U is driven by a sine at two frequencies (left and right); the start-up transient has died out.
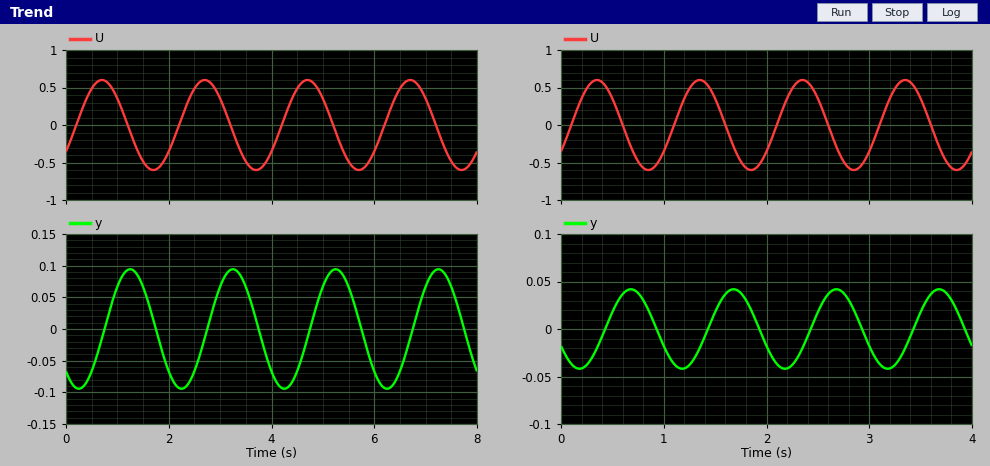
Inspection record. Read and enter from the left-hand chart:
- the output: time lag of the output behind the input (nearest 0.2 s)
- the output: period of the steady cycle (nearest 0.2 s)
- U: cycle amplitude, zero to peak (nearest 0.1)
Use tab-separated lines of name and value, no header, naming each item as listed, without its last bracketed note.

the output: time lag of the output behind the input	0.6 s
the output: period of the steady cycle	2.0 s
U: cycle amplitude, zero to peak	0.6
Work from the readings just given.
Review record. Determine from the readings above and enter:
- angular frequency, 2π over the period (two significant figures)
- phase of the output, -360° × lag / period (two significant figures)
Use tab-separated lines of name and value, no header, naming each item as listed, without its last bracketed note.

angular frequency, 2π over the period	3.1 rad/s
phase of the output, -360° × lag / period	-110°
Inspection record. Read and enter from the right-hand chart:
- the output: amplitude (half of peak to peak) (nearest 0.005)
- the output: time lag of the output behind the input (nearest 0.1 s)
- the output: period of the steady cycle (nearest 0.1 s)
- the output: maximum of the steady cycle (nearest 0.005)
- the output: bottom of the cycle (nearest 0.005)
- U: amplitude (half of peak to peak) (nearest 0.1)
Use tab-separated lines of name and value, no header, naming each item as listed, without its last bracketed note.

the output: amplitude (half of peak to peak)	0.040
the output: time lag of the output behind the input	0.3 s
the output: period of the steady cycle	1.0 s
the output: maximum of the steady cycle	0.040
the output: bottom of the cycle	-0.040
U: amplitude (half of peak to peak)	0.6
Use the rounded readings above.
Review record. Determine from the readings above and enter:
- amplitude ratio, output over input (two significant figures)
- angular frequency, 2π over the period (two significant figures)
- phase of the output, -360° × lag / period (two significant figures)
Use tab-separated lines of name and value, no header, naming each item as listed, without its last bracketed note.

amplitude ratio, output over input	0.067
angular frequency, 2π over the period	6.3 rad/s
phase of the output, -360° × lag / period	-110°
